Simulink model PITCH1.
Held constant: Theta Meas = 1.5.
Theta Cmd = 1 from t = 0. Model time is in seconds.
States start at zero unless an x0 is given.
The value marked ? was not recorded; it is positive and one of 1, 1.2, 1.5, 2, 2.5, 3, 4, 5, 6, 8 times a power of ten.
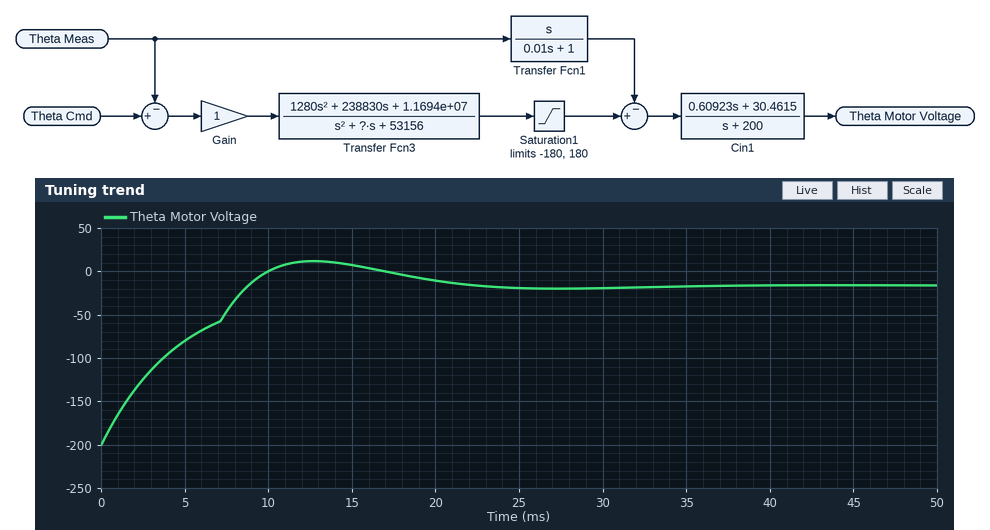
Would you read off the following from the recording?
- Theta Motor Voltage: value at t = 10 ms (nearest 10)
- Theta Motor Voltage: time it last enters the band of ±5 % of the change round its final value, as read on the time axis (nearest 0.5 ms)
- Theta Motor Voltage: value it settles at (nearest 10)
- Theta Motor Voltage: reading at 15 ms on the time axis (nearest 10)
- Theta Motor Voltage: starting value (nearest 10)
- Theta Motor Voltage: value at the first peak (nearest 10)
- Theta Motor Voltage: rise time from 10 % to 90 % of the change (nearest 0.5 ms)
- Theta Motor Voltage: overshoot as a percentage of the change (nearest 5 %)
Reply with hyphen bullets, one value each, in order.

- 0
- 19.0 ms
- -20
- 10
- -200
- 10
- 7.5 ms
- 15 %
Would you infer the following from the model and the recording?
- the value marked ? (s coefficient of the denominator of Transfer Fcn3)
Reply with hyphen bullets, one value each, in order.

- 300
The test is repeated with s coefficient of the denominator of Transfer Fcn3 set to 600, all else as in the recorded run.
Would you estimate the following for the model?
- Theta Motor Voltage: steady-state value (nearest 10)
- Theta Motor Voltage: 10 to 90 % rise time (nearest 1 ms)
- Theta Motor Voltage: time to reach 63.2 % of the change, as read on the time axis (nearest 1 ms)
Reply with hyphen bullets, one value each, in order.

- -20
- 6 ms
- 4 ms
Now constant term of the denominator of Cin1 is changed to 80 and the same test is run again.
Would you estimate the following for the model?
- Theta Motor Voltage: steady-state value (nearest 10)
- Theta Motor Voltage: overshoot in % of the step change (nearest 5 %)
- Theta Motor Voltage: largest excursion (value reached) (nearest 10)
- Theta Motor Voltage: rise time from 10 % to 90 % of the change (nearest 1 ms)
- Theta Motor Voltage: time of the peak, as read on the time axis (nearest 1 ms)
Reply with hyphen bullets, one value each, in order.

- -40
- 10 %
- -30
- 9 ms
- 15 ms
